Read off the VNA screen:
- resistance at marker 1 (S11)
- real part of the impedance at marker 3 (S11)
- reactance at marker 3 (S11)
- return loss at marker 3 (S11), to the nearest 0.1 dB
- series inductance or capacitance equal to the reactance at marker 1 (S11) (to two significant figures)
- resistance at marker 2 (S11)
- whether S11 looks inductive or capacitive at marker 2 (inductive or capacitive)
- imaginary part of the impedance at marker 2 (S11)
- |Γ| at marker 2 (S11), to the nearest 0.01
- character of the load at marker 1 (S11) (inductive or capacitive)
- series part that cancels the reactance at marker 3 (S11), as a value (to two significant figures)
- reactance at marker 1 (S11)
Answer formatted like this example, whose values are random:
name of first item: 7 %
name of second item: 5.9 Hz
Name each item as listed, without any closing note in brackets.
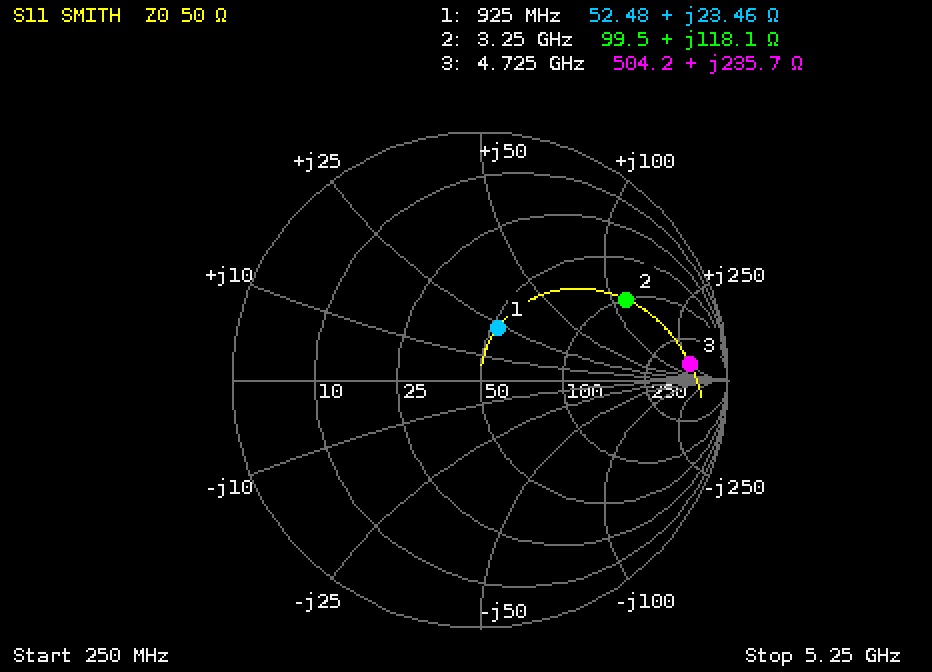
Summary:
resistance at marker 1: 52.48 Ω
real part of the impedance at marker 3: 504.2 Ω
reactance at marker 3: +235.7 Ω
return loss at marker 3 (S11), to the nearest 0.1 dB: 1.4 dB
series inductance or capacitance equal to the reactance at marker 1 (S11): 4.0 nH
resistance at marker 2: 99.5 Ω
whether S11 looks inductive or capacitive at marker 2: inductive
imaginary part of the impedance at marker 2: +118.1 Ω
|Γ| at marker 2 (S11), to the nearest 0.01: 0.67
character of the load at marker 1 (S11): inductive
series part that cancels the reactance at marker 3 (S11), as a value: 140 fF
reactance at marker 1: +23.46 Ω
